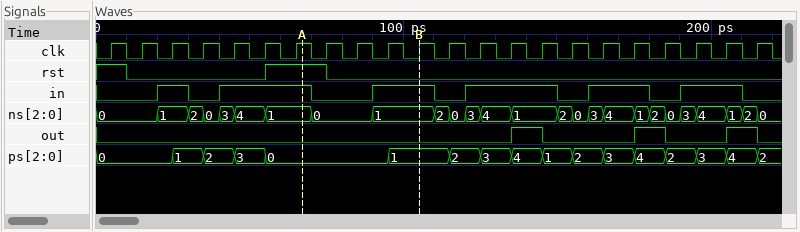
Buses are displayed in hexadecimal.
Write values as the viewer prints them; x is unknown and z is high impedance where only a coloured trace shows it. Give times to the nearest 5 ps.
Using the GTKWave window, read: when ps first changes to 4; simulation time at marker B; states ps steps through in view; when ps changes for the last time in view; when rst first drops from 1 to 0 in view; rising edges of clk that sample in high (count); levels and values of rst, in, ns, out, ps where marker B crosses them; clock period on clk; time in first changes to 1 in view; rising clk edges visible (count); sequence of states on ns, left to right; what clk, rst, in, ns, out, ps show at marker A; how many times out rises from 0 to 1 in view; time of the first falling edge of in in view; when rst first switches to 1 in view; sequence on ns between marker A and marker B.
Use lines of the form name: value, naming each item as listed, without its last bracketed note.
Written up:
when ps first changes to 4: 135 ps
simulation time at marker B: 105 ps
states ps steps through in view: 0, 1, 2, 3, 0, 1, 2, 3, 4, 1, 2, 3, 4, 2, 3, 4, 2
when ps changes for the last time in view: 215 ps
when rst first drops from 1 to 0 in view: 10 ps
rising edges of clk that sample in high: 13
levels and values of rst, in, ns, out, ps where marker B crosses them: rst=0, in=1, ns=1, out=0, ps=1
clock period on clk: 10 ps
time in first changes to 1 in view: 20 ps
rising clk edges visible: 22
sequence of states on ns, left to right: 0, 1, 2, 0, 3, 4, 1, 0, 1, 2, 0, 3, 4, 1, 2, 0, 3, 4, 1, 2, 0, 3, 4, 1, 2, 0
what clk, rst, in, ns, out, ps show at marker A: clk=1, rst=1, in=1, ns=1, out=0, ps=0
how many times out rises from 0 to 1 in view: 3
time of the first falling edge of in in view: 30 ps
when rst first switches to 1 in view: 55 ps
sequence on ns between marker A and marker B: 1, 0, 1
